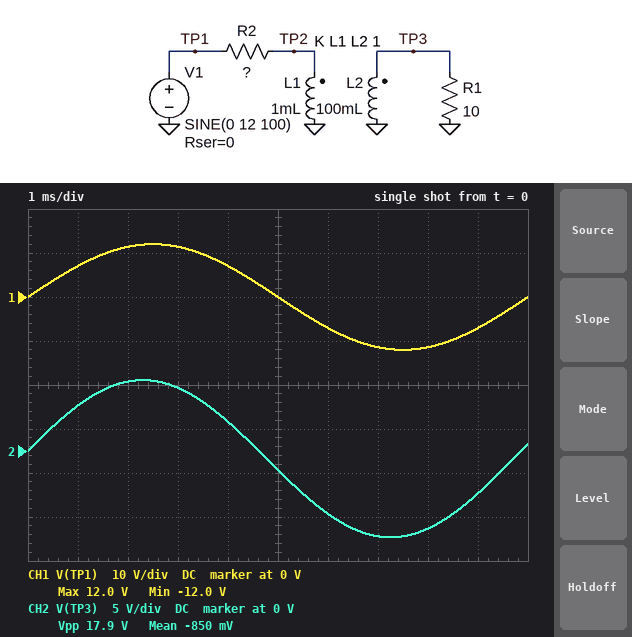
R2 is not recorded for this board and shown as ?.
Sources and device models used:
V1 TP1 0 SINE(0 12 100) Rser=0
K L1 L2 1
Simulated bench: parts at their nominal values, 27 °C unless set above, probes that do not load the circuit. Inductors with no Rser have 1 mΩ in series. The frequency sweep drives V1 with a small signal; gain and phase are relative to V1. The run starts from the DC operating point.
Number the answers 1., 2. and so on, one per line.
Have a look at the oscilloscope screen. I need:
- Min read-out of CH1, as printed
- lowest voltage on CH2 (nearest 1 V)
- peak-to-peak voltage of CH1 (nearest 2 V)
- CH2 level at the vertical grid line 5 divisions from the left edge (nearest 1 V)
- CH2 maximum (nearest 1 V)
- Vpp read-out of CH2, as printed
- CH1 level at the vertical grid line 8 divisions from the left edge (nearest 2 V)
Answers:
1. -12.0 V
2. -10 V
3. 24 V
4. -2 V
5. 8 V
6. 17.9 V
7. -12 V
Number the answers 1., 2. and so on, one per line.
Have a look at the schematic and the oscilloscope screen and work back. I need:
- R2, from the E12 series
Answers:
1. 1.2 Ω
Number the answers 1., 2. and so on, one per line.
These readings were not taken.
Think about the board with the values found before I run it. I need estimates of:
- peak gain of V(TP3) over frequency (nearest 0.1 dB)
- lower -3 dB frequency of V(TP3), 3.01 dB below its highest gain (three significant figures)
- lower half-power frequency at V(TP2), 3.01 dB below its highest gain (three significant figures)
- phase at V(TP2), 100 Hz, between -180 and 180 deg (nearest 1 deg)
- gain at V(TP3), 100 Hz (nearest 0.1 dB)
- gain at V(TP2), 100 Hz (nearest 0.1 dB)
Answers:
1. -2.3 dB
2. 14.7 Hz
3. 14.7 Hz
4. 8 deg
5. -2.4 dB
6. -22.3 dB
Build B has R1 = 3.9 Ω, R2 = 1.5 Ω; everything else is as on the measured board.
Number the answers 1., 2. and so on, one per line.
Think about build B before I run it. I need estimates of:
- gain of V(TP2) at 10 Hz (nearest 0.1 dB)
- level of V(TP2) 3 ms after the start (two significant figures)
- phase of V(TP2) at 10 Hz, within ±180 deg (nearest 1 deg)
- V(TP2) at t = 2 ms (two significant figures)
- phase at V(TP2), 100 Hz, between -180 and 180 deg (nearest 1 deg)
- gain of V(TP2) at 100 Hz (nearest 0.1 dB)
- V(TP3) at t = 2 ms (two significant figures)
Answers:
1. -33.1 dB
2. 270 mV
3. 30 deg
4. 280 mV
5. 3 deg
6. -31.7 dB
7. 2.8 V
